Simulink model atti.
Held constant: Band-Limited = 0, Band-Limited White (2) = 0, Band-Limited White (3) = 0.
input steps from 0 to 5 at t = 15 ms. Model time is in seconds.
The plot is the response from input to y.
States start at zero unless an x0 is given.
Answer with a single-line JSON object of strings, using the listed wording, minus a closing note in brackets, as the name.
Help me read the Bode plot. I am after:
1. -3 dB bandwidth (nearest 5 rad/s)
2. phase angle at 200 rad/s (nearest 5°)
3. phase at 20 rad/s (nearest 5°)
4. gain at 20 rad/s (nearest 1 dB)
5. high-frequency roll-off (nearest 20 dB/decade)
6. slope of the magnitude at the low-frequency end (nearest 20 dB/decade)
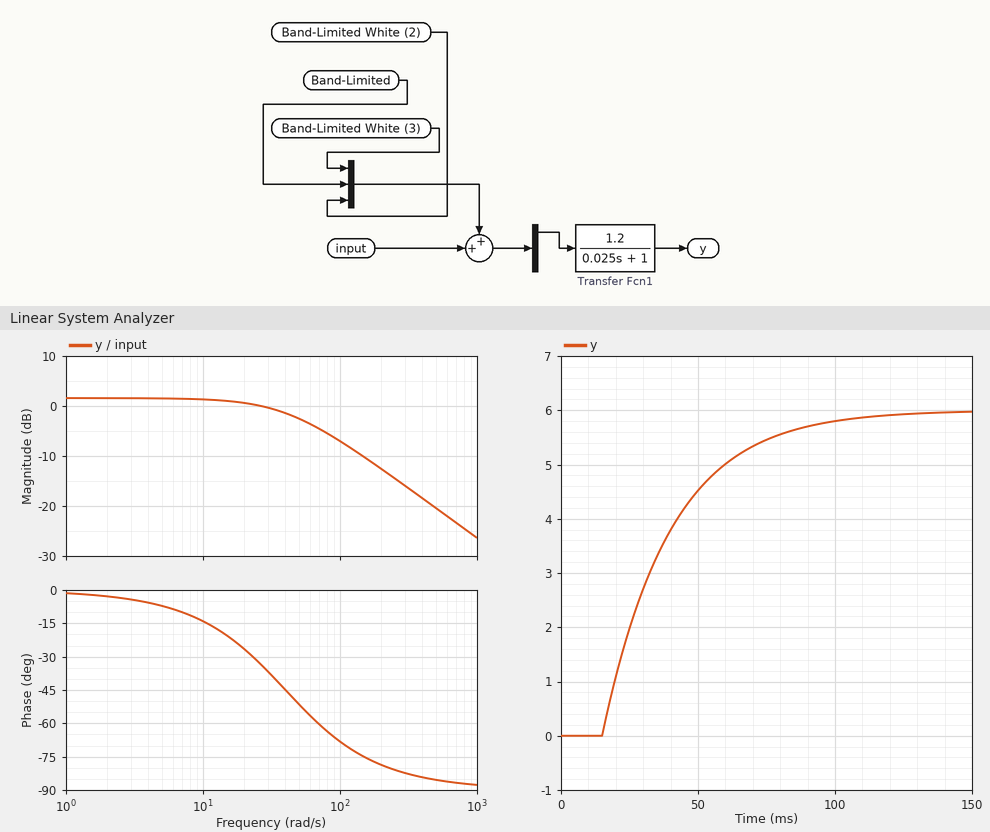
{"-3 dB bandwidth": "40 rad/s", "phase angle at 200 rad/s": "-80°", "phase at 20 rad/s": "-25°", "gain at 20 rad/s": "1 dB", "high-frequency roll-off": "-20 dB/decade", "slope of the magnitude at the low-frequency end": "0 dB/decade"}
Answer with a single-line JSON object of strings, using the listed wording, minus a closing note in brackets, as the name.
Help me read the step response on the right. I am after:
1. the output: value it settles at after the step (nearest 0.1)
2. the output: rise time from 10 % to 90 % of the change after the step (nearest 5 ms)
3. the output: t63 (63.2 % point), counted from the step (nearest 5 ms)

{"the output: value it settles at after the step": "6.0", "the output: rise time from 10 % to 90 % of the change after the step": "55 ms", "the output: t63 (63.2 % point), counted from the step": "25 ms"}
